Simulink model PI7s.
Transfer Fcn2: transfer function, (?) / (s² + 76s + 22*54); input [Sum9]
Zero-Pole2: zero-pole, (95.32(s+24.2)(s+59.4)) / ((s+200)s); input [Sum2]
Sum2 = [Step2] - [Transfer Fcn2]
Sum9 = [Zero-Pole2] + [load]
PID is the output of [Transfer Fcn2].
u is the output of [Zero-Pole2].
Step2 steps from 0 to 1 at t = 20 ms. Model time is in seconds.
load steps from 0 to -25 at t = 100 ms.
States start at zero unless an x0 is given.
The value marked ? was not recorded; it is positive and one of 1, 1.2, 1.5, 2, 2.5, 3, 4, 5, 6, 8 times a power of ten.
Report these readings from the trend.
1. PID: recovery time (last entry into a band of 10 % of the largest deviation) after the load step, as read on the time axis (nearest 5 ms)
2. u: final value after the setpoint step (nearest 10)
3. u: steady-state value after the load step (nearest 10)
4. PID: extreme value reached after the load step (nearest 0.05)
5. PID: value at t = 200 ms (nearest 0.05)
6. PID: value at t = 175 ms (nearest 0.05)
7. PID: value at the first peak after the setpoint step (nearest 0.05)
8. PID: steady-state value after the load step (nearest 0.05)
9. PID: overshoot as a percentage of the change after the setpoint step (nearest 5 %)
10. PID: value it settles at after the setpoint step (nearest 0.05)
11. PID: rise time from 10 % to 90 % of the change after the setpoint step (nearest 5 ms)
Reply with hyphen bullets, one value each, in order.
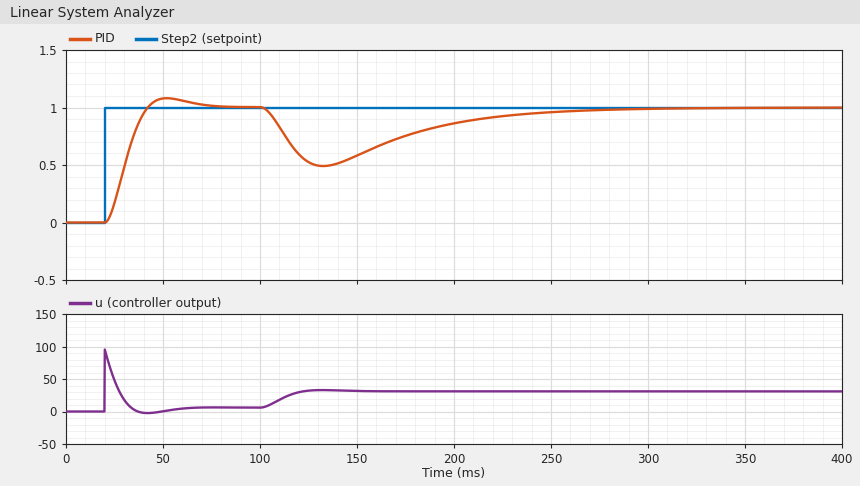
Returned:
- 240 ms
- 10
- 30
- 0.50
- 0.85
- 0.75
- 1.10
- 1.00
- 10 %
- 1.00
- 15 ms
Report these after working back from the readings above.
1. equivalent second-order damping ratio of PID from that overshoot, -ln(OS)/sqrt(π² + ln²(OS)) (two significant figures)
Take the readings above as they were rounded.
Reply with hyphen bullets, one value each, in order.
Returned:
- 0.59
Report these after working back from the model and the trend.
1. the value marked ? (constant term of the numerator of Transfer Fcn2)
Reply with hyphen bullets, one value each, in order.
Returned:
- 200
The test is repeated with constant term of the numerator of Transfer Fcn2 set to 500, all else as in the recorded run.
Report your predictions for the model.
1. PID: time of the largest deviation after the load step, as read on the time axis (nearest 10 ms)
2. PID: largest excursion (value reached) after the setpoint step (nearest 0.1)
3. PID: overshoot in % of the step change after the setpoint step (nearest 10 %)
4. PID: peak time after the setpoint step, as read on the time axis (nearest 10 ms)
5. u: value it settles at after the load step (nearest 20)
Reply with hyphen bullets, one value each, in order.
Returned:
- 120 ms
- 1.2
- 20 %
- 40 ms
- 20
